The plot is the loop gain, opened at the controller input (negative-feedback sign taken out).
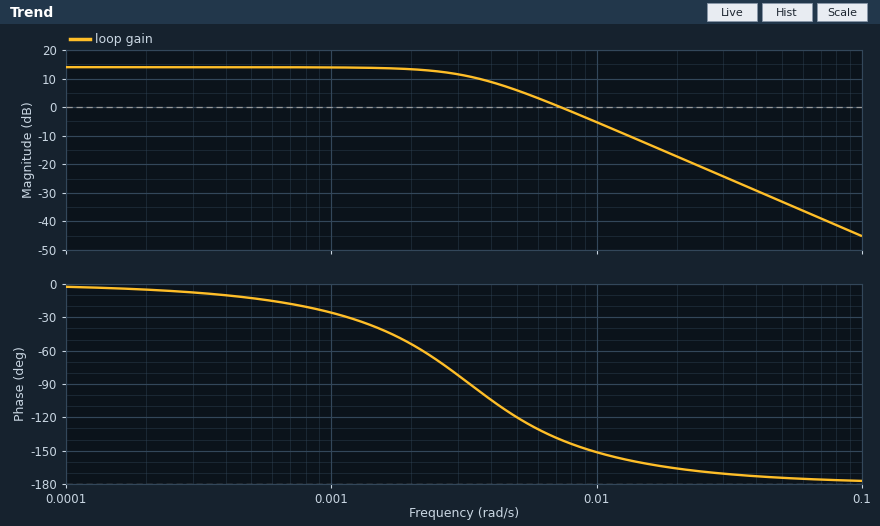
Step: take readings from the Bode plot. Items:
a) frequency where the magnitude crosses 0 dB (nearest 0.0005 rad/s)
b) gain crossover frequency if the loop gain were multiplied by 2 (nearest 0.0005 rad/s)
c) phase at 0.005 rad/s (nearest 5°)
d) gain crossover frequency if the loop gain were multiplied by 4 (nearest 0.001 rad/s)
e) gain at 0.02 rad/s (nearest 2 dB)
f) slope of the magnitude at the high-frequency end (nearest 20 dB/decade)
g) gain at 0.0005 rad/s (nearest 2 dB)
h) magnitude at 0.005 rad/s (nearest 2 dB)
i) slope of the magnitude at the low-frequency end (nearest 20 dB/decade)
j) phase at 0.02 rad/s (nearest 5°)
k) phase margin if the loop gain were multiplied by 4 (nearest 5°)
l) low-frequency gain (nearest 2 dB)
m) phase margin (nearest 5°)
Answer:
0.0075 rad/s
0.0105 rad/s
-120°
0.015 rad/s
-18 dB
-40 dB/decade
14 dB
6 dB
0 dB/decade
-165°
20°
14 dB
40°
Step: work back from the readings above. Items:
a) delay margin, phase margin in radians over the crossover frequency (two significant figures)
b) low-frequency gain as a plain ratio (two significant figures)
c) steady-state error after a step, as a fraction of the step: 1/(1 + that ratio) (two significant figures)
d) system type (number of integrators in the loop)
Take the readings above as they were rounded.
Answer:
93 s
5.0
0.17
0
